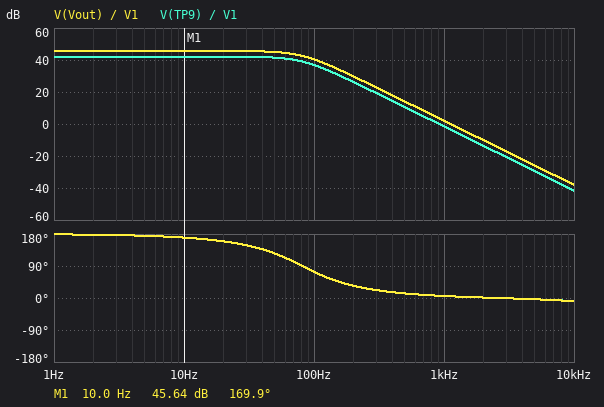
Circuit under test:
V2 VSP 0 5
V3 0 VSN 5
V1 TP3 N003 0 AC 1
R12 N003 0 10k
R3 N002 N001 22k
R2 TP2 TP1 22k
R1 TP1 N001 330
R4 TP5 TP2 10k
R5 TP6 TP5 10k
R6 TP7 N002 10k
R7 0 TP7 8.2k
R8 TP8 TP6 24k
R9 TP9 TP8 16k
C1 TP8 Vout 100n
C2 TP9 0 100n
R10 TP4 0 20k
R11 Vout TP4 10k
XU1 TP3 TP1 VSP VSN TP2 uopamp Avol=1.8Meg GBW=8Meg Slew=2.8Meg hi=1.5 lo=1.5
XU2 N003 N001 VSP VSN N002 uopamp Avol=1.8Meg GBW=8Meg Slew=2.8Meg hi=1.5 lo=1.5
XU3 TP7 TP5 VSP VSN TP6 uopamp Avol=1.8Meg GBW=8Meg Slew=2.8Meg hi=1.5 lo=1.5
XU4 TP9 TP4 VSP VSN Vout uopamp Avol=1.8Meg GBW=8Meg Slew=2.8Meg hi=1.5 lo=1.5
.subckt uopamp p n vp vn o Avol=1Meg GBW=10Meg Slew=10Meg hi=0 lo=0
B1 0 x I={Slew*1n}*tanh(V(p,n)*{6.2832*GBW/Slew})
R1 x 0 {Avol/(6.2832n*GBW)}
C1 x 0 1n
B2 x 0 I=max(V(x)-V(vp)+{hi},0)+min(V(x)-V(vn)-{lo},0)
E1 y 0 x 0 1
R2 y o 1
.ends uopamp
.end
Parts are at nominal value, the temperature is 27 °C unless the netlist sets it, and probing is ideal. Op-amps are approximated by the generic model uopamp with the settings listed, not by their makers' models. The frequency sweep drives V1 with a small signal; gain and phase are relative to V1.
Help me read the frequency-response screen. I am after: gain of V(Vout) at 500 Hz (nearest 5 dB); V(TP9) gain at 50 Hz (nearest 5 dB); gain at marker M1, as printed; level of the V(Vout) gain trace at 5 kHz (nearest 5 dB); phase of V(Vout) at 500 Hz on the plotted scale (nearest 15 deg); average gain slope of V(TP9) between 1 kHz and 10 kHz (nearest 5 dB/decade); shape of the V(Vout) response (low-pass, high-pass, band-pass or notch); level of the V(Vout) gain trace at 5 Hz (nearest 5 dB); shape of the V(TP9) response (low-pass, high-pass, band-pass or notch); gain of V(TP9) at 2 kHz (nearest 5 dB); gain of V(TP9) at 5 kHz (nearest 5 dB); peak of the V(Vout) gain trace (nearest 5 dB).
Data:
15 dB
40 dB
45.64 dB
-25 dB
15 deg
-40 dB/decade
low-pass
45 dB
low-pass
-15 dB
-30 dB
45 dB
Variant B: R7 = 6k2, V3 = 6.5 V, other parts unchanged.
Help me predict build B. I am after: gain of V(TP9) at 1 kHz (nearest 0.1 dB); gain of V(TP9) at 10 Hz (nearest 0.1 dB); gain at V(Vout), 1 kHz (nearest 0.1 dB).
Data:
-2.1 dB
41.5 dB
1.4 dB
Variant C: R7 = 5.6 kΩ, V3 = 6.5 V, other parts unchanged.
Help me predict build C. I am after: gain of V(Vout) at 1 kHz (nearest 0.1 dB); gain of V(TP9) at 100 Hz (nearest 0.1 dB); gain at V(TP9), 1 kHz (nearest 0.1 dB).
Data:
1.2 dB
36.0 dB
-2.4 dB
